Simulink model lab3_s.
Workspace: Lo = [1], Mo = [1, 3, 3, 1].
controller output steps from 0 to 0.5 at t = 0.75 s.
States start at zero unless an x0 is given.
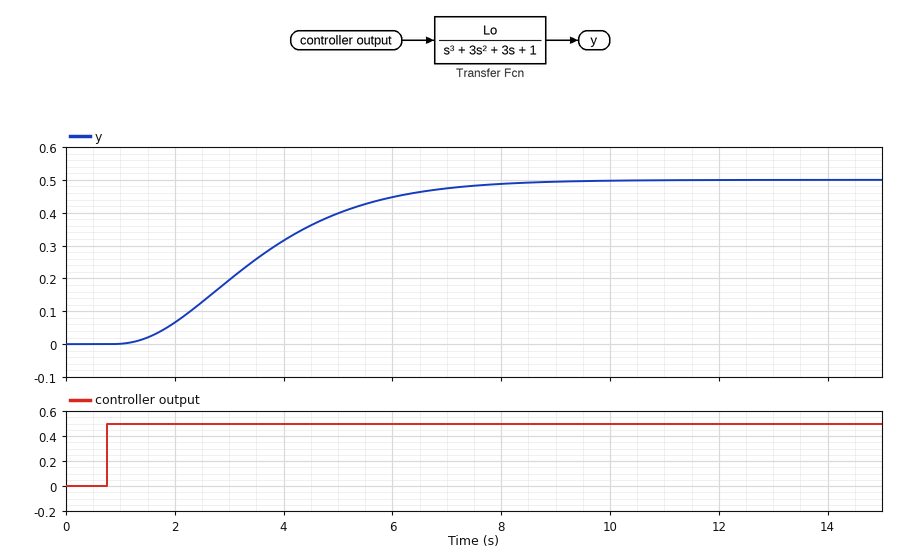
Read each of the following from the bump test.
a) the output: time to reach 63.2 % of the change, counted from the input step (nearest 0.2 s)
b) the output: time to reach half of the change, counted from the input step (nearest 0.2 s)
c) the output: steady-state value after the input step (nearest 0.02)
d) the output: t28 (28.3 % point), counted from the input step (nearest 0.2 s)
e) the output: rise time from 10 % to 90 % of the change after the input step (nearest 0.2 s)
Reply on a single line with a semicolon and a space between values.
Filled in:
3.2 s; 2.6 s; 0.50; 1.8 s; 4.2 s
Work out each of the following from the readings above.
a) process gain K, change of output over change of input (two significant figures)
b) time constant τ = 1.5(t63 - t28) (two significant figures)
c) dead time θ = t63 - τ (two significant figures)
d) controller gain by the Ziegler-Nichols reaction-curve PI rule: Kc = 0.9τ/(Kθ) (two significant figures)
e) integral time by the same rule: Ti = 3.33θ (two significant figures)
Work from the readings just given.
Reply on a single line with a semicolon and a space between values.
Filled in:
1.0; 2.1 s; 1.1 s; 1.7; 3.7 s
